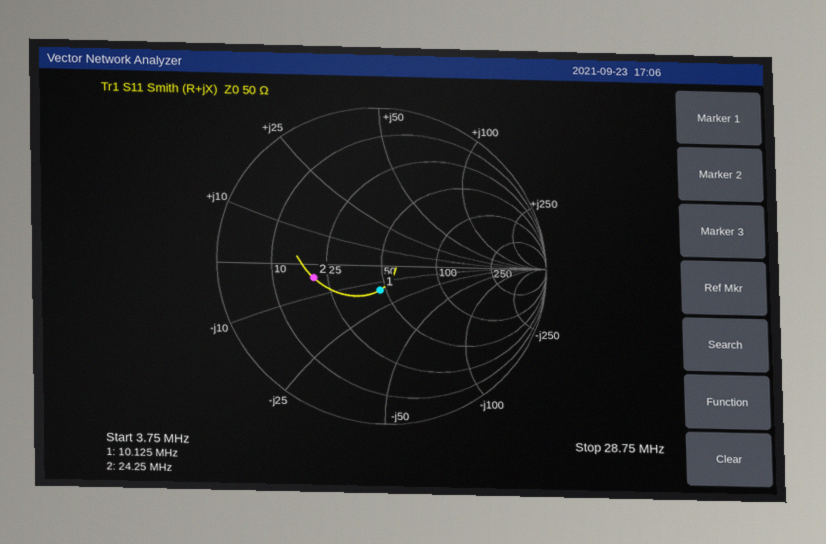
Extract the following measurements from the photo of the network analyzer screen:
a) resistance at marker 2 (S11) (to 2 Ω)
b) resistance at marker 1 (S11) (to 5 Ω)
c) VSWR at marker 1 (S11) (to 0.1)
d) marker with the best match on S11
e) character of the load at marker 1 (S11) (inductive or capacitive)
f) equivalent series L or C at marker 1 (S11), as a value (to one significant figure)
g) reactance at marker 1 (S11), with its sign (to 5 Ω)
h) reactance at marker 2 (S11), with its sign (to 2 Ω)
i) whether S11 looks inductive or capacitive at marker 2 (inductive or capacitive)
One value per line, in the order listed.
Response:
20 Ω
45 Ω
1.4
marker 1
capacitive
1 nF
-15 Ω
-4 Ω
capacitive
